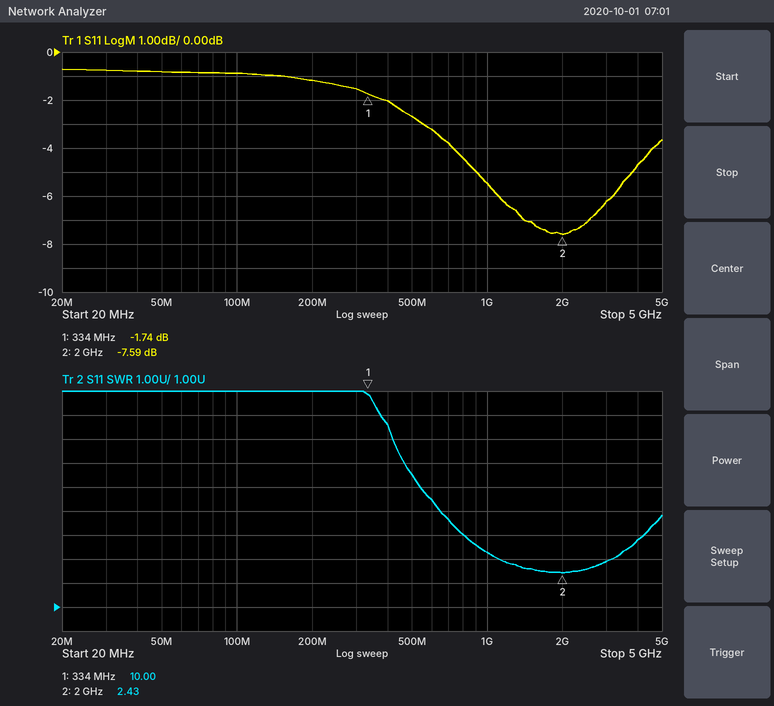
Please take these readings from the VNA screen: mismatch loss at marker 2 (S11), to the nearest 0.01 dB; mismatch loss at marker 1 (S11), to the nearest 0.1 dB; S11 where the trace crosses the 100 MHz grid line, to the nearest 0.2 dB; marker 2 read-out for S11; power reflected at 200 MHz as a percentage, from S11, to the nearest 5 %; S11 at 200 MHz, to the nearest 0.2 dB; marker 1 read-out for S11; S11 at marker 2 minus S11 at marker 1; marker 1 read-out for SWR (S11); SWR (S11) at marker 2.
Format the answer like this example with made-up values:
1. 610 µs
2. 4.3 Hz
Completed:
1. 0.83 dB
2. 4.8 dB
3. -0.8 dB
4. -7.59 dB
5. 75 %
6. -1.2 dB
7. -1.74 dB
8. -5.85 dB
9. 10.00
10. 2.43
